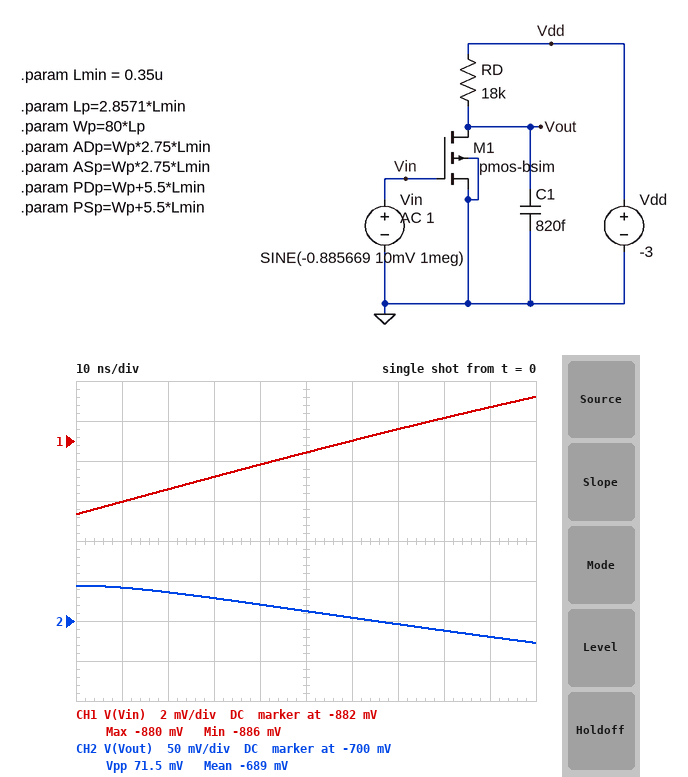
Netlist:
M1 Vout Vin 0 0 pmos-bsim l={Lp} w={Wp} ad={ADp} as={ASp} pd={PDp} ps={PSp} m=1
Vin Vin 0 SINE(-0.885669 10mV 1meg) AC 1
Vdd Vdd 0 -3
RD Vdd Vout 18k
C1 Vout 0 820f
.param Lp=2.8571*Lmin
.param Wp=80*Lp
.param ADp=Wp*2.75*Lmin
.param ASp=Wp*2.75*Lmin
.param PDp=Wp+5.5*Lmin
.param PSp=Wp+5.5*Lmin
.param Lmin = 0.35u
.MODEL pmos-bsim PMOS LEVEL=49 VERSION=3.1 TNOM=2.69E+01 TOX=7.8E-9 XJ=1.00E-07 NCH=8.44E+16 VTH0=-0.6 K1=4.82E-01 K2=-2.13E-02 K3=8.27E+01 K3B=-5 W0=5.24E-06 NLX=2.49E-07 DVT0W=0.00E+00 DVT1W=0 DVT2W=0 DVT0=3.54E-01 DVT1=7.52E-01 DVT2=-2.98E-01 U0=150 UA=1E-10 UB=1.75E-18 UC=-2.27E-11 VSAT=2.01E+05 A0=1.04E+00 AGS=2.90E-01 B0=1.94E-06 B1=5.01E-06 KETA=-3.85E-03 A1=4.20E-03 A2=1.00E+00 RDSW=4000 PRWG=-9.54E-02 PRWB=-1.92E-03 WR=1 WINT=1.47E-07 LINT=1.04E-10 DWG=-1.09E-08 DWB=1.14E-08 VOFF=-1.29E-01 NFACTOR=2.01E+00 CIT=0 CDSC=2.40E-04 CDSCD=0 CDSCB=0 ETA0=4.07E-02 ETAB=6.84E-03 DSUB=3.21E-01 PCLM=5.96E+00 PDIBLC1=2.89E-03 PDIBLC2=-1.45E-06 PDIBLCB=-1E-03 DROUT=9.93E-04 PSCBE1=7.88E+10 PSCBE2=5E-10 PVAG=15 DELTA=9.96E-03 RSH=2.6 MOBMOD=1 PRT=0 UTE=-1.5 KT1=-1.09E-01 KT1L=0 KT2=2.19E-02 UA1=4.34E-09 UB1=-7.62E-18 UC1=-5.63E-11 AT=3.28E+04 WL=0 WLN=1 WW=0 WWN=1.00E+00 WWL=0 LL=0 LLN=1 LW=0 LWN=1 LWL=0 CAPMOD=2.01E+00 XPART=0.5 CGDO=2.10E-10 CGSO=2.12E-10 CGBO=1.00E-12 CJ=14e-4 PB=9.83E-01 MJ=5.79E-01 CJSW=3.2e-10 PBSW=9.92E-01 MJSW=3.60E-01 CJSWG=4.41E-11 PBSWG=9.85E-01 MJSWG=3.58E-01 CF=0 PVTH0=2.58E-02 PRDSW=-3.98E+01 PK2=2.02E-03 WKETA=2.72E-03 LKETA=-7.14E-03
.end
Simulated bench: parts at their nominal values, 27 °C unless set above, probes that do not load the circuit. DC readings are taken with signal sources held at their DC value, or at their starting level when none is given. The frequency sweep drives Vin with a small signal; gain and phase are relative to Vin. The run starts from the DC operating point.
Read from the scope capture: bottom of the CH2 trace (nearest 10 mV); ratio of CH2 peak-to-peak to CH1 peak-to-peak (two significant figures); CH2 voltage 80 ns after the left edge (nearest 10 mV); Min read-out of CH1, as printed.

-730 mV
12
-710 mV
-886 mV
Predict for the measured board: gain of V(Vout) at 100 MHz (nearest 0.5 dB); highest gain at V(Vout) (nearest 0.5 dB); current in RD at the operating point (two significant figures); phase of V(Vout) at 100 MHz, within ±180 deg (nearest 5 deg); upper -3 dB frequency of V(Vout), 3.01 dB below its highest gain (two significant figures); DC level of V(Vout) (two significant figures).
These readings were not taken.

4.5 dB
23.0 dB
130 µA
90 deg
12 MHz
-660 mV
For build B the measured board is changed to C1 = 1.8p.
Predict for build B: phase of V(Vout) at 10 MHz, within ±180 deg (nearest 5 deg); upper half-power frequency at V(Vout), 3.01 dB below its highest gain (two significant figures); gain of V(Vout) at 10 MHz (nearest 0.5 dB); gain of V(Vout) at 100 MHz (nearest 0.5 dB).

120 deg
6.0 MHz
17.0 dB
-1.5 dB
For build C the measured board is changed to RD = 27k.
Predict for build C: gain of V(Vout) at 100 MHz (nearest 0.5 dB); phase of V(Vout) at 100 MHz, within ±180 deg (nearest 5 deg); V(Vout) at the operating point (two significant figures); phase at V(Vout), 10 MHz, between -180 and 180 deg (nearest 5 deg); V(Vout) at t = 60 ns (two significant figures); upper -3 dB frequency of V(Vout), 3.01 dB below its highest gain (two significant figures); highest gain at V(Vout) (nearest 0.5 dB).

-0.5 dB
110 deg
-160 mV
170 deg
-170 mV
57 MHz
5.5 dB
